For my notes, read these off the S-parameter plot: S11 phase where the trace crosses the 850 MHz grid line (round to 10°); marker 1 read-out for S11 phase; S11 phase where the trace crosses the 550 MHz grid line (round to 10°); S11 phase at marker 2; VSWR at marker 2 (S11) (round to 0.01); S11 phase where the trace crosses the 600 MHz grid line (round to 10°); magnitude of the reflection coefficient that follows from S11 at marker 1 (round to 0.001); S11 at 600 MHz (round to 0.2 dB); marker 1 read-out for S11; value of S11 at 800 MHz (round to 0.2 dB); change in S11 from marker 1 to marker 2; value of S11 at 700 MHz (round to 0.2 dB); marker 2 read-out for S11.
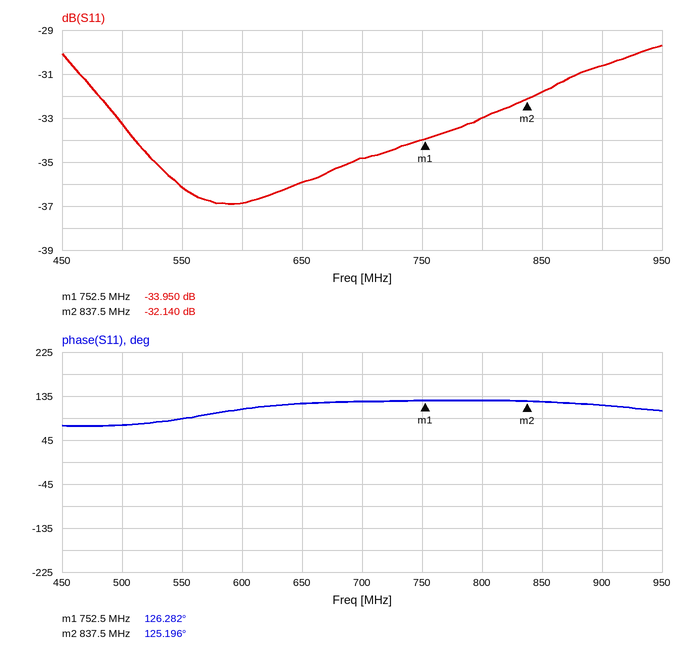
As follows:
120°
126.282°
90°
125.196°
1.05
110°
0.020
-36.8 dB
-33.950 dB
-33.0 dB
1.810 dB
-34.8 dB
-32.140 dB
